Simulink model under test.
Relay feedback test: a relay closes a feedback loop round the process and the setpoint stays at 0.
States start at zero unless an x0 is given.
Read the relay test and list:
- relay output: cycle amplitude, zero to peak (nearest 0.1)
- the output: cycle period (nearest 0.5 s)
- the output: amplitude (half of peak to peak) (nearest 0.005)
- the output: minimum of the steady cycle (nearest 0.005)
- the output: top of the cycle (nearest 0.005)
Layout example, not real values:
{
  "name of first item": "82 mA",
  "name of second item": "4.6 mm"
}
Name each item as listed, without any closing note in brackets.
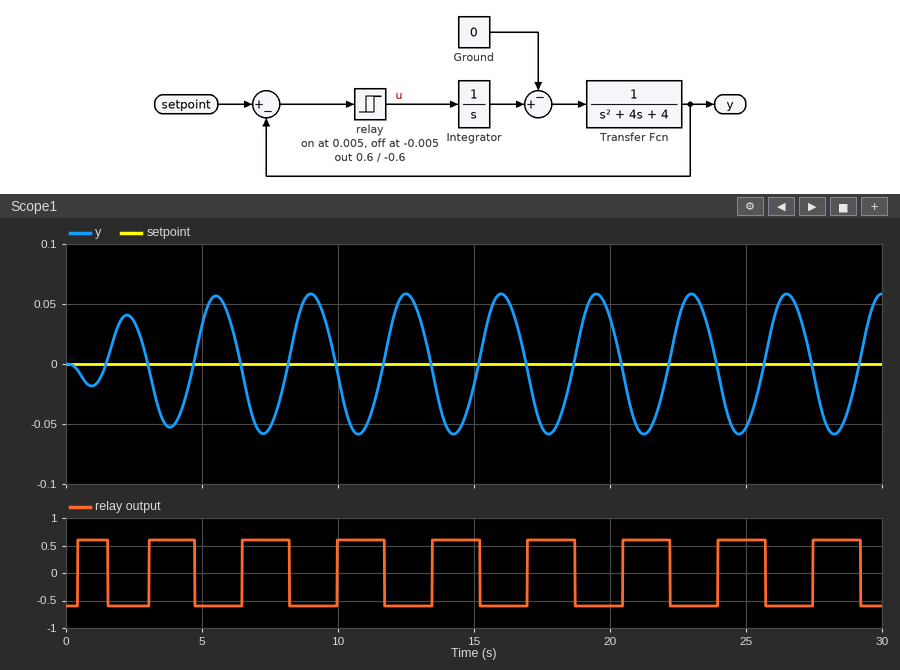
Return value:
{
  "relay output: cycle amplitude, zero to peak": "0.6",
  "the output: cycle period": "3.5 s",
  "the output: amplitude (half of peak to peak)": "0.060",
  "the output: minimum of the steady cycle": "-0.060",
  "the output: top of the cycle": "0.060"
}
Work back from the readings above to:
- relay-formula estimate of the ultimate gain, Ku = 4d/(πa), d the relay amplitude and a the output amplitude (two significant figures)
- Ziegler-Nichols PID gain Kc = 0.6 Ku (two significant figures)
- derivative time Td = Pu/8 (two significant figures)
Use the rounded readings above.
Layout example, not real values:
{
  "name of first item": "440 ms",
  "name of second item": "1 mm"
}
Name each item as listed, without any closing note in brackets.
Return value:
{
  "relay-formula estimate of the ultimate gain, Ku = 4d/(πa), d the relay amplitude and a the output amplitude": "13",
  "Ziegler-Nichols PID gain Kc = 0.6 Ku": "7.8",
  "derivative time Td = Pu/8": "0.44 s"
}
